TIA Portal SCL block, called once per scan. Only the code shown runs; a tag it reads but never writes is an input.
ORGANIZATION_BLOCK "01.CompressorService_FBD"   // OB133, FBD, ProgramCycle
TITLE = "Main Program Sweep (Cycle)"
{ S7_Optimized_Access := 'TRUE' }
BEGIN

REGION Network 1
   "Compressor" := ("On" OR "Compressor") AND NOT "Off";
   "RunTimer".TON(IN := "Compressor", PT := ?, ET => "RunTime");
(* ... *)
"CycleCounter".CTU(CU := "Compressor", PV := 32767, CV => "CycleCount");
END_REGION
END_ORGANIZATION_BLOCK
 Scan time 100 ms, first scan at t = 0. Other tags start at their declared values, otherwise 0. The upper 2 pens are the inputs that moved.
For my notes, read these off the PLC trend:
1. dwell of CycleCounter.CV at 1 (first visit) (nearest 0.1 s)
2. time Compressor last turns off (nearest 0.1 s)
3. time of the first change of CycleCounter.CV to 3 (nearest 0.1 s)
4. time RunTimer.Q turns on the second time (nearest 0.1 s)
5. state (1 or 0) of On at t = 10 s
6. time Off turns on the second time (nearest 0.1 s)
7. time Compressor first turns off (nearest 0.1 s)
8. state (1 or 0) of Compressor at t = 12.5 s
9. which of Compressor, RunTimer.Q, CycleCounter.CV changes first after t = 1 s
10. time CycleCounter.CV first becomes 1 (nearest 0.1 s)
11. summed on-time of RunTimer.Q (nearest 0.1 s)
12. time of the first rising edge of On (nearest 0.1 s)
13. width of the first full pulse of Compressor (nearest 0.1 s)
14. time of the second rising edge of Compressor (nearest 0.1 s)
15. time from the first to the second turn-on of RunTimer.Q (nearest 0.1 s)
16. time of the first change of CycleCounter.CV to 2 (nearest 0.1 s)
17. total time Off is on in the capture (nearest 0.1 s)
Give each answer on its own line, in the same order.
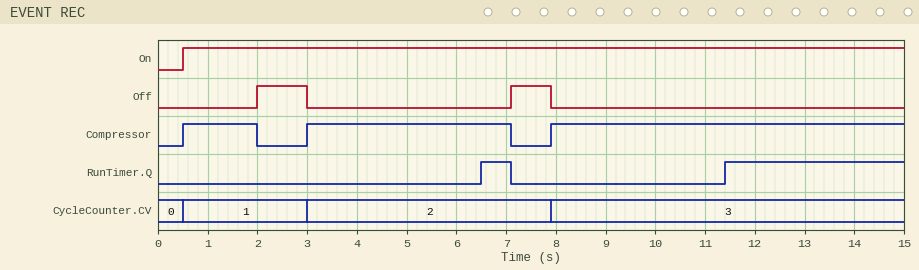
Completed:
2.5 s
7.1 s
7.9 s
11.4 s
1
7.1 s
2.0 s
1
Compressor
0.5 s
4.2 s
0.5 s
1.5 s
3.0 s
4.9 s
3.0 s
1.8 s
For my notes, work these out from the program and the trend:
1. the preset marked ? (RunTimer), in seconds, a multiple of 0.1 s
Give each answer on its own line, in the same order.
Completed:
3.5 s
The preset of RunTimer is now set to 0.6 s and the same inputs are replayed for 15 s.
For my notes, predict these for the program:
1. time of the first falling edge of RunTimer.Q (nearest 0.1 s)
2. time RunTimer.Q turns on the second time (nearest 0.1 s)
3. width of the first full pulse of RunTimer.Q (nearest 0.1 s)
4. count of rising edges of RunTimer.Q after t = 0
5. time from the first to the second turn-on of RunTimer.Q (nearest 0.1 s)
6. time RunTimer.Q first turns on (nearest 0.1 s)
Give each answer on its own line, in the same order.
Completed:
2.0 s
3.6 s
0.9 s
3
2.5 s
1.1 s
